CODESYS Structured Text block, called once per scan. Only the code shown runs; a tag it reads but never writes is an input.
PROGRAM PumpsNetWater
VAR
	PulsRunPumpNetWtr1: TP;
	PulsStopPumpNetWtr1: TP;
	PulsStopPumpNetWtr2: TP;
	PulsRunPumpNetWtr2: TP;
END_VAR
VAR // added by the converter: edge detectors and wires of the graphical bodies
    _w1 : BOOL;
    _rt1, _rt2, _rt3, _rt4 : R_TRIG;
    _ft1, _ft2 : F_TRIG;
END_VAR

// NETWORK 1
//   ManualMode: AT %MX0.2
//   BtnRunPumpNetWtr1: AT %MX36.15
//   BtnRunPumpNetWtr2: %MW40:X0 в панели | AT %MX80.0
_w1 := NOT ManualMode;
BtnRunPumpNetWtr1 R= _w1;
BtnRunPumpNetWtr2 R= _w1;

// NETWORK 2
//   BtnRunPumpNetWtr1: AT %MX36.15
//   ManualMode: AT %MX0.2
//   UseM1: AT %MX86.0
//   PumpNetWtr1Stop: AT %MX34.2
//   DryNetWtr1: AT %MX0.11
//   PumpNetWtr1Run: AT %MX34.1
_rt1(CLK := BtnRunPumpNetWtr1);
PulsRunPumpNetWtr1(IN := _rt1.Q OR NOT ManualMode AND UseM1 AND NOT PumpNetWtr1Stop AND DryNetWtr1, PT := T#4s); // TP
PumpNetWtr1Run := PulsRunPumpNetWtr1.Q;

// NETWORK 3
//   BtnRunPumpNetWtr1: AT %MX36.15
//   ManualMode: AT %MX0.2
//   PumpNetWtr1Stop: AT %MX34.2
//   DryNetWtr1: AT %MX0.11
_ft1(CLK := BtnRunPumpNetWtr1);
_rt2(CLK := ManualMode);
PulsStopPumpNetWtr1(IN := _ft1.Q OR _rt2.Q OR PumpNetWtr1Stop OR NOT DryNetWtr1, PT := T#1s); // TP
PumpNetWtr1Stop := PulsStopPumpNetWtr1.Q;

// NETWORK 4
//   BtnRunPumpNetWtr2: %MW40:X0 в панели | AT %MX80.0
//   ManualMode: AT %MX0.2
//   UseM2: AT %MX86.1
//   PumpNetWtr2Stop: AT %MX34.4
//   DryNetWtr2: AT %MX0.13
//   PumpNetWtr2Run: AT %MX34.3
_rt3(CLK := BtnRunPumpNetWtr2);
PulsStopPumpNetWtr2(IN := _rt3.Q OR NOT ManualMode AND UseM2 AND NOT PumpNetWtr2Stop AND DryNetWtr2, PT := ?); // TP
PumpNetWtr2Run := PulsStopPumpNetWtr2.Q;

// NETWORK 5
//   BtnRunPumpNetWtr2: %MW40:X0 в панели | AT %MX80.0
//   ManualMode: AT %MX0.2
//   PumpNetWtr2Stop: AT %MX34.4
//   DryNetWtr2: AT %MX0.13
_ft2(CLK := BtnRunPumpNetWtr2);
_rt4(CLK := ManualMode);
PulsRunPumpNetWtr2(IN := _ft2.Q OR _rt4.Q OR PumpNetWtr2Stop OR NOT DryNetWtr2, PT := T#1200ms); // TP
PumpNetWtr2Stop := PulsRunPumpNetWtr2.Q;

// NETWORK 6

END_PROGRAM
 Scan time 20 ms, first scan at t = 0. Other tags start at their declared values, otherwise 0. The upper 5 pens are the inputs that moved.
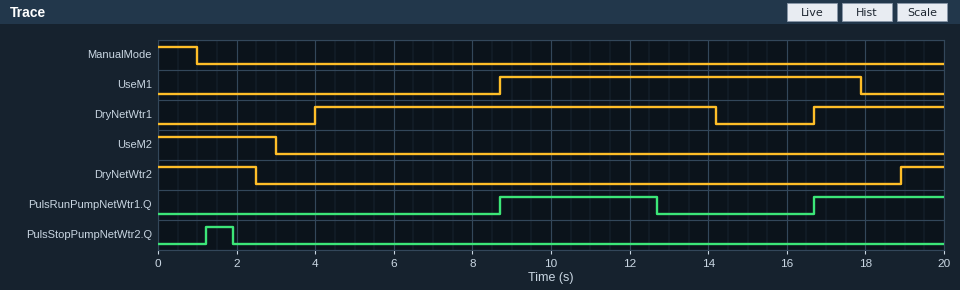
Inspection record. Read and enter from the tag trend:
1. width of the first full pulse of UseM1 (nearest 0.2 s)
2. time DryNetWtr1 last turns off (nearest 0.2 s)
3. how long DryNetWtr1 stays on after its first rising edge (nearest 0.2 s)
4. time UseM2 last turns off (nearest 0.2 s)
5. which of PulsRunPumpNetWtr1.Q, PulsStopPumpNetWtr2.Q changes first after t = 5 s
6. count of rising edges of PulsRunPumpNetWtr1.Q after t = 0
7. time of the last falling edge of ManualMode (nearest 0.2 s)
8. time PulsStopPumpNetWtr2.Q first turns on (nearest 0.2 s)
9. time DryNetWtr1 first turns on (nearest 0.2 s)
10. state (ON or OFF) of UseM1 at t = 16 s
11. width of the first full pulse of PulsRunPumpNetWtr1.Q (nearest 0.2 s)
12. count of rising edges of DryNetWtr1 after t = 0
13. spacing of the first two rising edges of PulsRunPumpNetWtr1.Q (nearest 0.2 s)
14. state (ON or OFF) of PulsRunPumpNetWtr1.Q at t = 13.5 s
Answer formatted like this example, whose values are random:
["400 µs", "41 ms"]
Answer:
["9.2 s", "14.2 s", "10.2 s", "3.0 s", "PulsRunPumpNetWtr1.Q", "2", "1.0 s", "1.2 s", "4.0 s", "ON", "4.0 s", "2", "8.0 s", "OFF"]
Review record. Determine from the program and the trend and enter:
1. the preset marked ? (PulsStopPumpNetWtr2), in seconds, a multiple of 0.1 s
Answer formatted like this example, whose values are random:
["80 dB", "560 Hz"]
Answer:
["0.7 s"]
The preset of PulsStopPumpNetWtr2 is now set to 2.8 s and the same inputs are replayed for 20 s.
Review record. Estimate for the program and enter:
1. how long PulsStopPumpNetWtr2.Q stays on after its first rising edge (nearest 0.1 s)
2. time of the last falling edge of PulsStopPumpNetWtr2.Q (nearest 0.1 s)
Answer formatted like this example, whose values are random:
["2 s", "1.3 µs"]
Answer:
["2.8 s", "4.0 s"]
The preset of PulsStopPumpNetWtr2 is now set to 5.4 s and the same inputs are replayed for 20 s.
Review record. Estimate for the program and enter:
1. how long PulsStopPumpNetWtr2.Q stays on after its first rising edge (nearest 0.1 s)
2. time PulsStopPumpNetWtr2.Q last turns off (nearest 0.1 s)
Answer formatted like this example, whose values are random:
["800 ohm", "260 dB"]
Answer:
["5.4 s", "6.6 s"]
